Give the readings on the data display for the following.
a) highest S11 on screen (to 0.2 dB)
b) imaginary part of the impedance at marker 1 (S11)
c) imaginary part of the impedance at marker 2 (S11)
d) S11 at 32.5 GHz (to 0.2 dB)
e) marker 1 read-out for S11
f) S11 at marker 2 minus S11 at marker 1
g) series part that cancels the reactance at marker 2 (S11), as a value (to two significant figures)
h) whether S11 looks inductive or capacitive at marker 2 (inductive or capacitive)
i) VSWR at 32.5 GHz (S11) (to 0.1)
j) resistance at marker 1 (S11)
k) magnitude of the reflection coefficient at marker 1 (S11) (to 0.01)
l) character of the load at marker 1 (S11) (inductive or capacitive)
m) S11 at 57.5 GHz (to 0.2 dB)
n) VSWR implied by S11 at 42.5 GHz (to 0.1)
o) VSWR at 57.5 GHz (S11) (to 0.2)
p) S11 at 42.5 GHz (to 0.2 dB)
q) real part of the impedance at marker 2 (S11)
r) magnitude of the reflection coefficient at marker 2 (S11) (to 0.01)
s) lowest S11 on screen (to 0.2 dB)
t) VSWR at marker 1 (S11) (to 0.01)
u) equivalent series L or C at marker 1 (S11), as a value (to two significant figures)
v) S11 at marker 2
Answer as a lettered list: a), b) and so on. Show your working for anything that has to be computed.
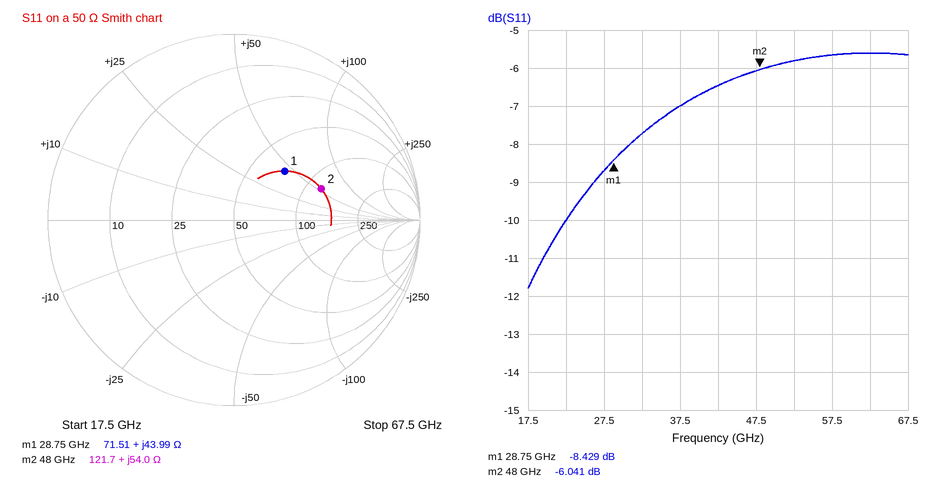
a) -5.6 dB
b) +43.99 Ω
c) +54.0 Ω
d) -7.8 dB
e) -8.429 dB
f) -6.041 − (-8.429) = 2.388 dB
g) C = 1/(2π × 48 GHz × 54 Ω) ≈ 61 fF
h) inductive
i) |Γ| = 10^(-7.8/20) = 0.4074; VSWR = (1 + 0.4074)/(1 − 0.4074) ≈ 2.4
j) 71.51 Ω
k) 0.38
l) inductive
m) -5.6 dB
n) |Γ| = 10^(-6.4/20) = 0.4786; VSWR = (1 + 0.4786)/(1 − 0.4786) ≈ 2.8
o) |Γ| = 10^(-5.6/20) = 0.5248; VSWR = (1 + 0.5248)/(1 − 0.5248) ≈ 3.2
p) -6.4 dB
q) 121.7 Ω
r) 10^(-6.041/20) ≈ 0.50
s) -11.8 dB
t) (1 + 0.3789)/(1 − 0.3789) ≈ 2.22
u) L = 43.99 Ω/(2π × 28.75 GHz) ≈ 244 pH, so 240 pH to two significant figures
v) -6.041 dB
